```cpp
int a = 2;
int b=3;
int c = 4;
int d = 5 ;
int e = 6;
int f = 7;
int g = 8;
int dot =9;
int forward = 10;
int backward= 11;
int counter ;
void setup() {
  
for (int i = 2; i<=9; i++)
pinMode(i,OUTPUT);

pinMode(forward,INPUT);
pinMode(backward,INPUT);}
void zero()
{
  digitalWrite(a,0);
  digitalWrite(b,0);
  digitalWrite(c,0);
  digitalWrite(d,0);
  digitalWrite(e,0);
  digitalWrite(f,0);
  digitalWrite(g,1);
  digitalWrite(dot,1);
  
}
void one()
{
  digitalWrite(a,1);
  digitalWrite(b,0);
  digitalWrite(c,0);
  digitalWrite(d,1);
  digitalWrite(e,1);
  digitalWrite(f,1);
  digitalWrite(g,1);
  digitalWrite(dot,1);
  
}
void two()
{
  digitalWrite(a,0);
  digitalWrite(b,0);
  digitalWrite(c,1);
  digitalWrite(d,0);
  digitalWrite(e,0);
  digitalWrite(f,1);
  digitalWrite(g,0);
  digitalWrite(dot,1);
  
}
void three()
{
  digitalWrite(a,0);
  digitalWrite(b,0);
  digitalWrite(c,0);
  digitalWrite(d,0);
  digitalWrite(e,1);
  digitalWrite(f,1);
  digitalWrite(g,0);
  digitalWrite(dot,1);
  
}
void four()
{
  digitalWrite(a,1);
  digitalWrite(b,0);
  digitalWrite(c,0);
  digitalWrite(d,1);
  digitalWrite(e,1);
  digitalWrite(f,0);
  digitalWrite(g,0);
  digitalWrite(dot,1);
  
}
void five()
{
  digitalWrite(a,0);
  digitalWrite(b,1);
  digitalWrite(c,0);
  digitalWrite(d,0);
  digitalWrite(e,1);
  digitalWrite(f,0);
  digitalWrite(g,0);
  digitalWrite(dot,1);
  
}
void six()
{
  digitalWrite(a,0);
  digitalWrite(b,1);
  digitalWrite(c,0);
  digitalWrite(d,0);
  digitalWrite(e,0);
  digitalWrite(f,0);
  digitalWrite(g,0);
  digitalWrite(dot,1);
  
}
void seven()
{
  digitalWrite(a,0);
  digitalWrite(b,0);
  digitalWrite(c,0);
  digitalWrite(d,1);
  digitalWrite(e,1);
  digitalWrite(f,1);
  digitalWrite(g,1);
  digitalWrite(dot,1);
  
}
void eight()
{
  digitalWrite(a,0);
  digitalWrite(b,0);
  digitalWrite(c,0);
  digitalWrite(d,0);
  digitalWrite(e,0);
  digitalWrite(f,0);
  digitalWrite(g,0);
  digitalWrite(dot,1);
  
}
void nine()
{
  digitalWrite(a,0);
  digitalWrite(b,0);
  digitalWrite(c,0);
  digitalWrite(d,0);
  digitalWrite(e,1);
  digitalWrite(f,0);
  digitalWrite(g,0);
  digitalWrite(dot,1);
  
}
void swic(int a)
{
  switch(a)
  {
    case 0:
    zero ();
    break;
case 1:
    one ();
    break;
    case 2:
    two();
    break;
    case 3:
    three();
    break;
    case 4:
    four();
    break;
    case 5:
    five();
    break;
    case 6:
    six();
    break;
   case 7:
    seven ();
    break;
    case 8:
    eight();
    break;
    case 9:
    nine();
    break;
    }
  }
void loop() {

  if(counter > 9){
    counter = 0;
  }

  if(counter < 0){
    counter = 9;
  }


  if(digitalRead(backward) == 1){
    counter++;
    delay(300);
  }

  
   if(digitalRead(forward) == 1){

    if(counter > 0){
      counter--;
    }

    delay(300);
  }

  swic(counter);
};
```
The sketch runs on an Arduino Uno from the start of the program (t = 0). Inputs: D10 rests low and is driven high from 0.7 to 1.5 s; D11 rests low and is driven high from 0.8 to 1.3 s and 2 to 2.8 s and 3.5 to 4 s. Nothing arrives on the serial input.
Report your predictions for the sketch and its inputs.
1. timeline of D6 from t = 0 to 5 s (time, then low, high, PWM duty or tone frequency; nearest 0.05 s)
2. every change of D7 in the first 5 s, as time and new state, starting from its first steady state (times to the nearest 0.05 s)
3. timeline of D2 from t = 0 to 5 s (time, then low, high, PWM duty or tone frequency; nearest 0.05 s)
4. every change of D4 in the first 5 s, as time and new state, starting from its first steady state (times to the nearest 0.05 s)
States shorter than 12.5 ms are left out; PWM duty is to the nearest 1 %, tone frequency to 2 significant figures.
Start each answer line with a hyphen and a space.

- 0 s low; 2.3 s high; 2.6 s low; 2.9 s high
- 0 s low; 2.3 s high; 3.8 s low
- 0 s low; 2.3 s high; 2.6 s low; 3.8 s high; 4.1 s low
- 0 s low; 2.6 s high; 2.9 s low
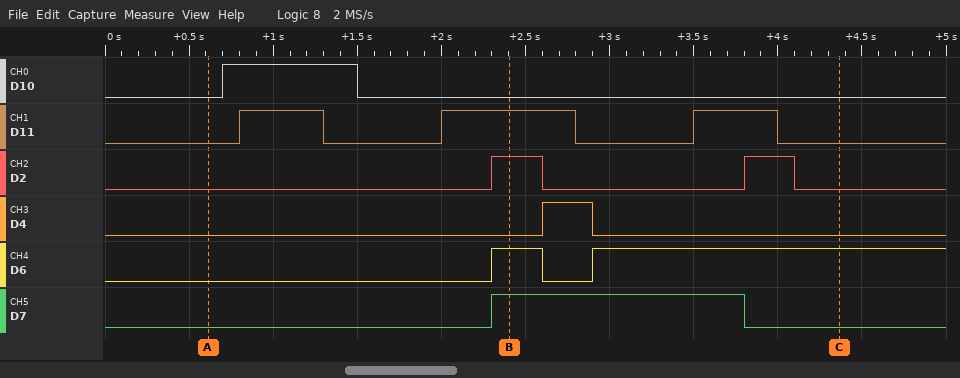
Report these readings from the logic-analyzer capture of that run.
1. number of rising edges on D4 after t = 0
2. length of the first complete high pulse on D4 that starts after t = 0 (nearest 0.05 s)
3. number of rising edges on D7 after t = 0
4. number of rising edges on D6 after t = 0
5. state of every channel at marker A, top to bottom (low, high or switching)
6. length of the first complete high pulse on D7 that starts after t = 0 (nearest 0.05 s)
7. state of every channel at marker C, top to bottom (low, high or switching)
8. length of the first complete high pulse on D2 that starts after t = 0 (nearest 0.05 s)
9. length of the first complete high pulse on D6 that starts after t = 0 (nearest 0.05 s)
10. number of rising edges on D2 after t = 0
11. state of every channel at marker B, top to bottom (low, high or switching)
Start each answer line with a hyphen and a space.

- 1
- 0.30 s
- 1
- 2
- D10 low, D11 low, D2 low, D4 low, D6 low, D7 low
- 1.50 s
- D10 low, D11 low, D2 low, D4 low, D6 high, D7 low
- 0.30 s
- 0.30 s
- 2
- D10 low, D11 high, D2 high, D4 low, D6 high, D7 high
